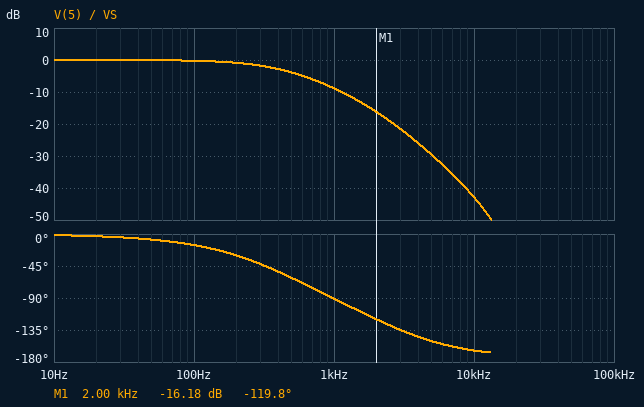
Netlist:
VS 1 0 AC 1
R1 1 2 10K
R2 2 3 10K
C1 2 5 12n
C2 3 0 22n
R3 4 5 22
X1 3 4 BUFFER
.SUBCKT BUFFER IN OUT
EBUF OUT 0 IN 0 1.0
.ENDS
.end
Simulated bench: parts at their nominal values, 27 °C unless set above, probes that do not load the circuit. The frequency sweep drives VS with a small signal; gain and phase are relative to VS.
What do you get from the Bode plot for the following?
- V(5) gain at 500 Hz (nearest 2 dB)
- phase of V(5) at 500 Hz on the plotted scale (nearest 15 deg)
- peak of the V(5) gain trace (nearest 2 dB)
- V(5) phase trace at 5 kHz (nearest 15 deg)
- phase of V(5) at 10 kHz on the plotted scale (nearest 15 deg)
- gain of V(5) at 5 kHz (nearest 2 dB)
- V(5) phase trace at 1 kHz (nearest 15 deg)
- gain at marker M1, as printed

-4 dB
-60 deg
0 dB
-150 deg
-165 deg
-30 dB
-90 deg
-16.18 dB
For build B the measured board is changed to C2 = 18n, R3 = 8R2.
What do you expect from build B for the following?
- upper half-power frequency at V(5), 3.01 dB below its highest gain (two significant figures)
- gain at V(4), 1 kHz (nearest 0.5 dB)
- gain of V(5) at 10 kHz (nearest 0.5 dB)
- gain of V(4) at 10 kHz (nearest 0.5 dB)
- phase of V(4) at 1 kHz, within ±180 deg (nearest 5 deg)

530 Hz
-7.0 dB
-39.5 dB
-39.0 dB
-85 deg
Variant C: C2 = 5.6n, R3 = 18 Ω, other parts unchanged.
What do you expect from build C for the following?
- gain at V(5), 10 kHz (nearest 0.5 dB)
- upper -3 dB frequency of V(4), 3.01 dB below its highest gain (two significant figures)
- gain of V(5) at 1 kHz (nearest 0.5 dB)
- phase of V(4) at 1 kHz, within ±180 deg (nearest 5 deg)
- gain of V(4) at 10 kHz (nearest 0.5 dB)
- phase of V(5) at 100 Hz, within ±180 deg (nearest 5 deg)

-29.0 dB
2.0 kHz
0 dB
-45 deg
-28.5 dB
-5 deg
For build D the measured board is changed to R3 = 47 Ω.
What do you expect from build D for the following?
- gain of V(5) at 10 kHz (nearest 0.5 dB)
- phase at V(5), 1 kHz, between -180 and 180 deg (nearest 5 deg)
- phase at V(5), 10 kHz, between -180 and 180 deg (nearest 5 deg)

-46.5 dB
-90 deg
-160 deg
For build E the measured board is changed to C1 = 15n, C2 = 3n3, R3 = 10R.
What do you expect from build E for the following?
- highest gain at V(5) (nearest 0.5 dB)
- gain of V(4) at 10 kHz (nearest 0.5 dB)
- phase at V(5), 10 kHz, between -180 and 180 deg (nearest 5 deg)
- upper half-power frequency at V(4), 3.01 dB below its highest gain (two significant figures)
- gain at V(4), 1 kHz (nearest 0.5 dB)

1.5 dB
-25.5 dB
-165 deg
2.7 kHz
1.0 dB
